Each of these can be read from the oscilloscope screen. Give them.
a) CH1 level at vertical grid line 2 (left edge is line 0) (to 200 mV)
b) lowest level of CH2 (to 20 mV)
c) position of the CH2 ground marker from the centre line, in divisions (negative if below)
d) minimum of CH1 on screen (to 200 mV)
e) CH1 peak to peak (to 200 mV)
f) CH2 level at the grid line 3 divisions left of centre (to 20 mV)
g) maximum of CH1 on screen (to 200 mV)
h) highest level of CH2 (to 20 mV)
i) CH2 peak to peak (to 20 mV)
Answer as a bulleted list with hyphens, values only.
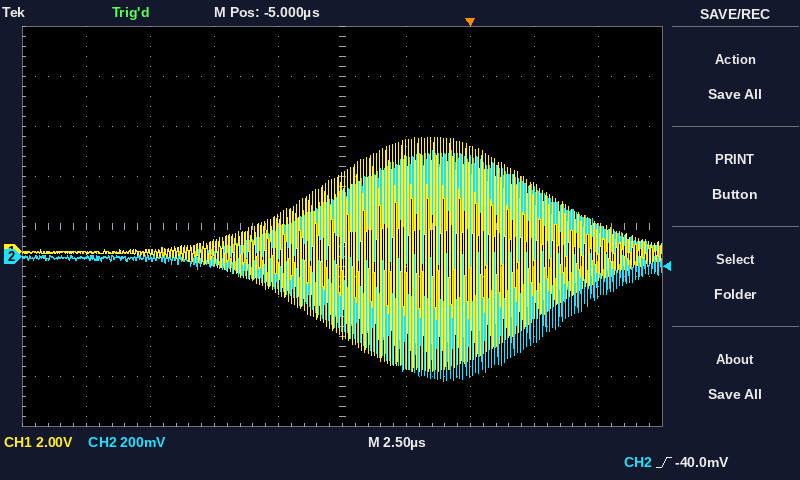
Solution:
- 0.0 V
- -500 mV
- -0.6 div
- -4.8 V
- 9.4 V
- 0 mV
- 4.6 V
- 420 mV
- 920 mV
